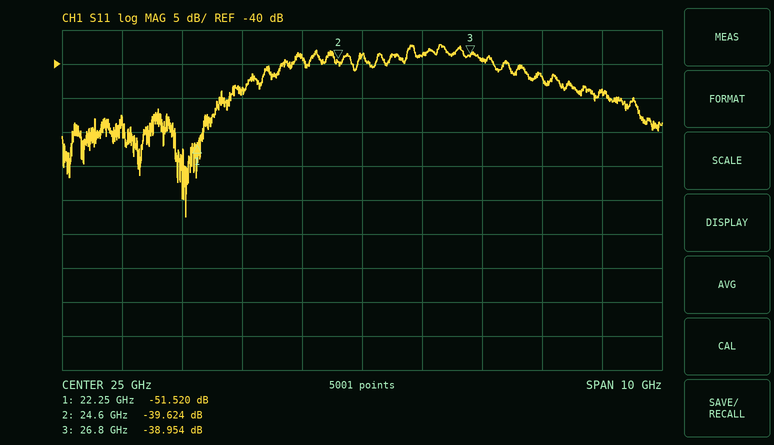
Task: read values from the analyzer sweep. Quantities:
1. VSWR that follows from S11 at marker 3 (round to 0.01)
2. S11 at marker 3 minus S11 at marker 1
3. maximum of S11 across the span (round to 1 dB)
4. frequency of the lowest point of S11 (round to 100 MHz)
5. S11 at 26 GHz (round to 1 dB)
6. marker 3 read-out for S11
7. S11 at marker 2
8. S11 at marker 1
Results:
1.02
12.566 dB
-37 dB
22.1 GHz
-39 dB
-38.954 dB
-39.624 dB
-51.520 dB
